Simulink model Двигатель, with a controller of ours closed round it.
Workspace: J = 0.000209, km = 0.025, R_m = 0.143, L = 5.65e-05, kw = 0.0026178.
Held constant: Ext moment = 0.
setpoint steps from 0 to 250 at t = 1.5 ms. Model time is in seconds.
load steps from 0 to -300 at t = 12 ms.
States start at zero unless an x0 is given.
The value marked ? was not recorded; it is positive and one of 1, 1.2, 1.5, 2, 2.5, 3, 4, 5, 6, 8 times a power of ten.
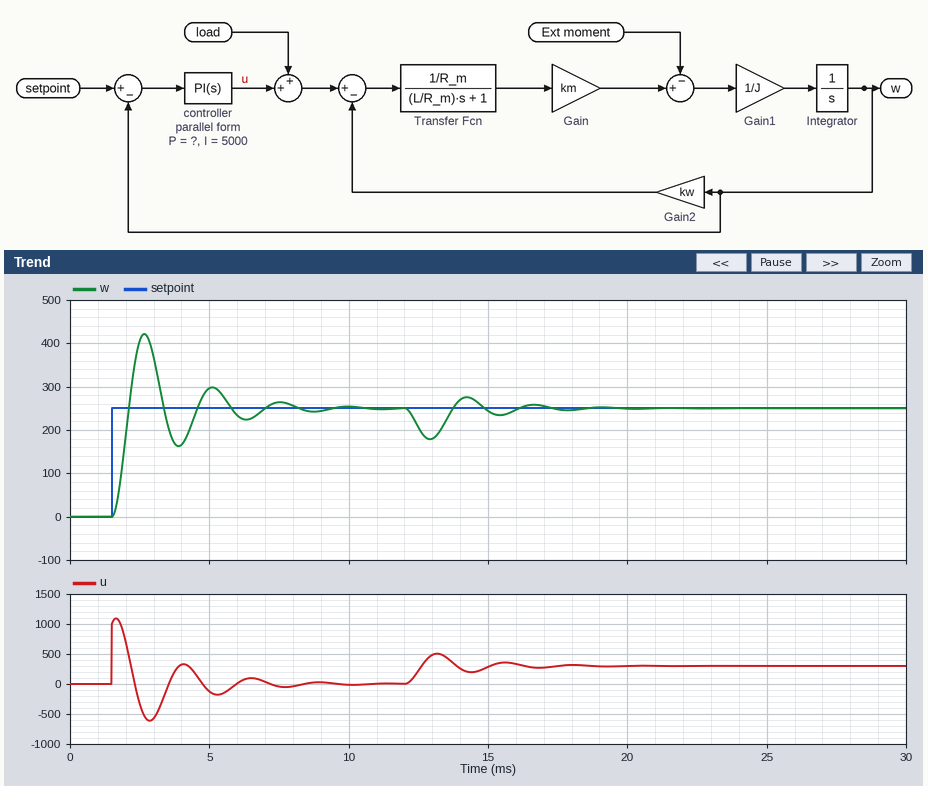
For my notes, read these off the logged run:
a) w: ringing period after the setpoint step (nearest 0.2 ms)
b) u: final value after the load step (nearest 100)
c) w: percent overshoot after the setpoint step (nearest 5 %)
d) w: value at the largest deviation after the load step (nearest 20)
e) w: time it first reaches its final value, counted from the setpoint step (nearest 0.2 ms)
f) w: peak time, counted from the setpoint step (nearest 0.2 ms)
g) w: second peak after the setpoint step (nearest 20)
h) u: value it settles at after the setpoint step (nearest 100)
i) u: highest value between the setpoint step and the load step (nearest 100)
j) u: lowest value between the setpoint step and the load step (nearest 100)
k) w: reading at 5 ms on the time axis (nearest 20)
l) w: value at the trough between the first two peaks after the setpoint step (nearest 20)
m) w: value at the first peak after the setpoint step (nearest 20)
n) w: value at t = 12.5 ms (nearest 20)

2.4 ms
300
70 %
180
0.6 ms
1.2 ms
300
0
1100
-600
300
160
420
200
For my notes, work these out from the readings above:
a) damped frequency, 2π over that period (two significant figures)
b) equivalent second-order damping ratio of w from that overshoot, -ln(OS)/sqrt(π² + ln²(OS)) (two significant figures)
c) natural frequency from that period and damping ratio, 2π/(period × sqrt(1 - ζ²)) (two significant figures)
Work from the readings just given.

2.6 rad/ms
0.11
2.6 rad/ms
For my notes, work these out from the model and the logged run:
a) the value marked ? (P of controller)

4
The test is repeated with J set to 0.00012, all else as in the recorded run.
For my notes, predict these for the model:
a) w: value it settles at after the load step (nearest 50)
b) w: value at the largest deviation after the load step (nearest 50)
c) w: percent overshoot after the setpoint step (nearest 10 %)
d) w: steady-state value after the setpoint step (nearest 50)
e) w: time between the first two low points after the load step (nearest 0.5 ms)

250
150
70 %
250
2.0 ms
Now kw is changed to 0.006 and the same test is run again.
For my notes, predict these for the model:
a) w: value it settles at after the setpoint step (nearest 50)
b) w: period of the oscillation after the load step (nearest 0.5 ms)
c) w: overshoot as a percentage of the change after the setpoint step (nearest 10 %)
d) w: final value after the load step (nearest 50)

250
2.5 ms
70 %
250
